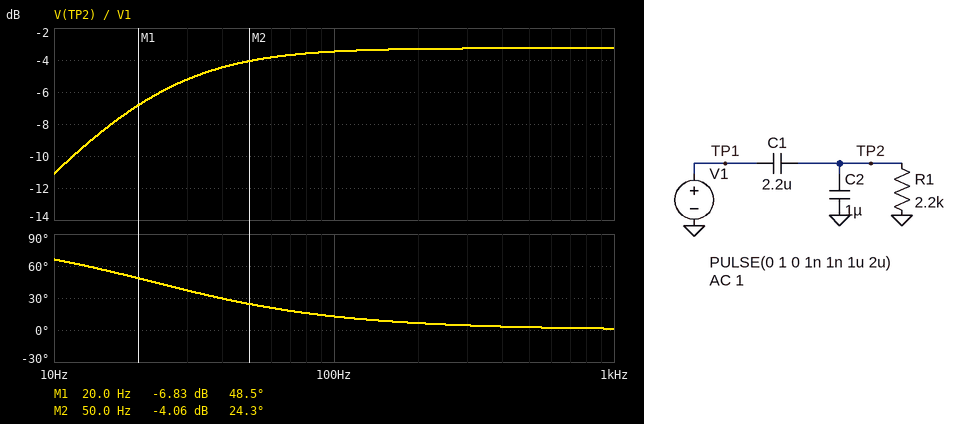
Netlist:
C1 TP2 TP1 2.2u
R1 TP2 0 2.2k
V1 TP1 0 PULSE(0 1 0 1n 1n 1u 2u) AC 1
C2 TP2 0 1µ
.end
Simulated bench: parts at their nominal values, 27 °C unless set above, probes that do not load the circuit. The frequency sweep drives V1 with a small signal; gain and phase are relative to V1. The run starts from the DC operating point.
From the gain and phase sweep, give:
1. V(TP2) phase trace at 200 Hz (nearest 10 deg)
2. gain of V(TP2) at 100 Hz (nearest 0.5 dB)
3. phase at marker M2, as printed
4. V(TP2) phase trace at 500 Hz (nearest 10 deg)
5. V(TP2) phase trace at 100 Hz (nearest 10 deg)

10 deg
-3.5 dB
24.3 deg
0 deg
10 deg
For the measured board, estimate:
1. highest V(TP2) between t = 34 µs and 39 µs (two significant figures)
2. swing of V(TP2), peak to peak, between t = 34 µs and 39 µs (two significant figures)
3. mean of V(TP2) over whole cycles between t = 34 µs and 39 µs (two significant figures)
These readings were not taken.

690 mV
690 mV
340 mV
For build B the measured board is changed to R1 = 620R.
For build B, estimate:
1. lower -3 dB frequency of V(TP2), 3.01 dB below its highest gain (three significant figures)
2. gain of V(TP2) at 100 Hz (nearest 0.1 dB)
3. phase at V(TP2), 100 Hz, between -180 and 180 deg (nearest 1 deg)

80.2 Hz
-5.4 dB
39 deg
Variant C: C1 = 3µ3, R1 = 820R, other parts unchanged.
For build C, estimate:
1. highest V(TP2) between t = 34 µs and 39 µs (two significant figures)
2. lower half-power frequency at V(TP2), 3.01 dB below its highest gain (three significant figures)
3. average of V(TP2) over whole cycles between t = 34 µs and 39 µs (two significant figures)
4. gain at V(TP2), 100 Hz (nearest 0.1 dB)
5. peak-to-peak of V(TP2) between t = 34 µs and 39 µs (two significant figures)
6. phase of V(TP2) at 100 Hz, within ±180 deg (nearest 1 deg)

760 mV
45.1 Hz
380 mV
-3.1 dB
770 mV
24 deg
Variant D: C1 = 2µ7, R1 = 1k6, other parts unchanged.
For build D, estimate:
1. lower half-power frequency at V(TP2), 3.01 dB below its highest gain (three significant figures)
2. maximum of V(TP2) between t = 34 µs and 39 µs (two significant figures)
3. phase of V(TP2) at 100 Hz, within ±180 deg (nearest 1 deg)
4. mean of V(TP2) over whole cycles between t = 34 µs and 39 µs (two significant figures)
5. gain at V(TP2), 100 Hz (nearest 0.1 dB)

26.9 Hz
730 mV
15 deg
360 mV
-3.0 dB
